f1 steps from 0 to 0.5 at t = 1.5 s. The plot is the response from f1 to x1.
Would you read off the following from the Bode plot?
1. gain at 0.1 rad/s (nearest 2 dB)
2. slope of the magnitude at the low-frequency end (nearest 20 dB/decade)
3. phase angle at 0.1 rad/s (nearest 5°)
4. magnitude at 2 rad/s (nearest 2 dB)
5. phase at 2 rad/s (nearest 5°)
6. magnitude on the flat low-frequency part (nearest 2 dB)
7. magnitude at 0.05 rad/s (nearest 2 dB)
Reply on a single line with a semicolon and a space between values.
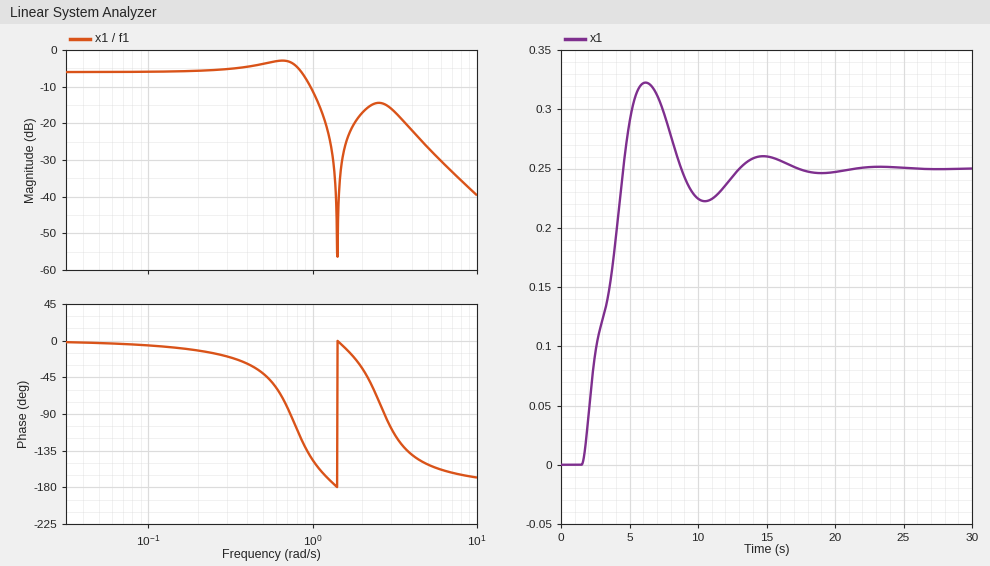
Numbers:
-6 dB; 0 dB/decade; -5°; -18 dB; -35°; -6 dB; -6 dB
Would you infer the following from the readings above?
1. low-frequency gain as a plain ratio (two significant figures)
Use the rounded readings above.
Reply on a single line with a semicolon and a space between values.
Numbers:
0.50
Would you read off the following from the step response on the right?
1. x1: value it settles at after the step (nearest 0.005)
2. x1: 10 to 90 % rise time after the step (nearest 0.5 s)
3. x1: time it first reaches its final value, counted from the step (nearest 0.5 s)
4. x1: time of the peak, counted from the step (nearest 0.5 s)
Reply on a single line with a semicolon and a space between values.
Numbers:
0.250; 2.5 s; 3.0 s; 4.5 s
